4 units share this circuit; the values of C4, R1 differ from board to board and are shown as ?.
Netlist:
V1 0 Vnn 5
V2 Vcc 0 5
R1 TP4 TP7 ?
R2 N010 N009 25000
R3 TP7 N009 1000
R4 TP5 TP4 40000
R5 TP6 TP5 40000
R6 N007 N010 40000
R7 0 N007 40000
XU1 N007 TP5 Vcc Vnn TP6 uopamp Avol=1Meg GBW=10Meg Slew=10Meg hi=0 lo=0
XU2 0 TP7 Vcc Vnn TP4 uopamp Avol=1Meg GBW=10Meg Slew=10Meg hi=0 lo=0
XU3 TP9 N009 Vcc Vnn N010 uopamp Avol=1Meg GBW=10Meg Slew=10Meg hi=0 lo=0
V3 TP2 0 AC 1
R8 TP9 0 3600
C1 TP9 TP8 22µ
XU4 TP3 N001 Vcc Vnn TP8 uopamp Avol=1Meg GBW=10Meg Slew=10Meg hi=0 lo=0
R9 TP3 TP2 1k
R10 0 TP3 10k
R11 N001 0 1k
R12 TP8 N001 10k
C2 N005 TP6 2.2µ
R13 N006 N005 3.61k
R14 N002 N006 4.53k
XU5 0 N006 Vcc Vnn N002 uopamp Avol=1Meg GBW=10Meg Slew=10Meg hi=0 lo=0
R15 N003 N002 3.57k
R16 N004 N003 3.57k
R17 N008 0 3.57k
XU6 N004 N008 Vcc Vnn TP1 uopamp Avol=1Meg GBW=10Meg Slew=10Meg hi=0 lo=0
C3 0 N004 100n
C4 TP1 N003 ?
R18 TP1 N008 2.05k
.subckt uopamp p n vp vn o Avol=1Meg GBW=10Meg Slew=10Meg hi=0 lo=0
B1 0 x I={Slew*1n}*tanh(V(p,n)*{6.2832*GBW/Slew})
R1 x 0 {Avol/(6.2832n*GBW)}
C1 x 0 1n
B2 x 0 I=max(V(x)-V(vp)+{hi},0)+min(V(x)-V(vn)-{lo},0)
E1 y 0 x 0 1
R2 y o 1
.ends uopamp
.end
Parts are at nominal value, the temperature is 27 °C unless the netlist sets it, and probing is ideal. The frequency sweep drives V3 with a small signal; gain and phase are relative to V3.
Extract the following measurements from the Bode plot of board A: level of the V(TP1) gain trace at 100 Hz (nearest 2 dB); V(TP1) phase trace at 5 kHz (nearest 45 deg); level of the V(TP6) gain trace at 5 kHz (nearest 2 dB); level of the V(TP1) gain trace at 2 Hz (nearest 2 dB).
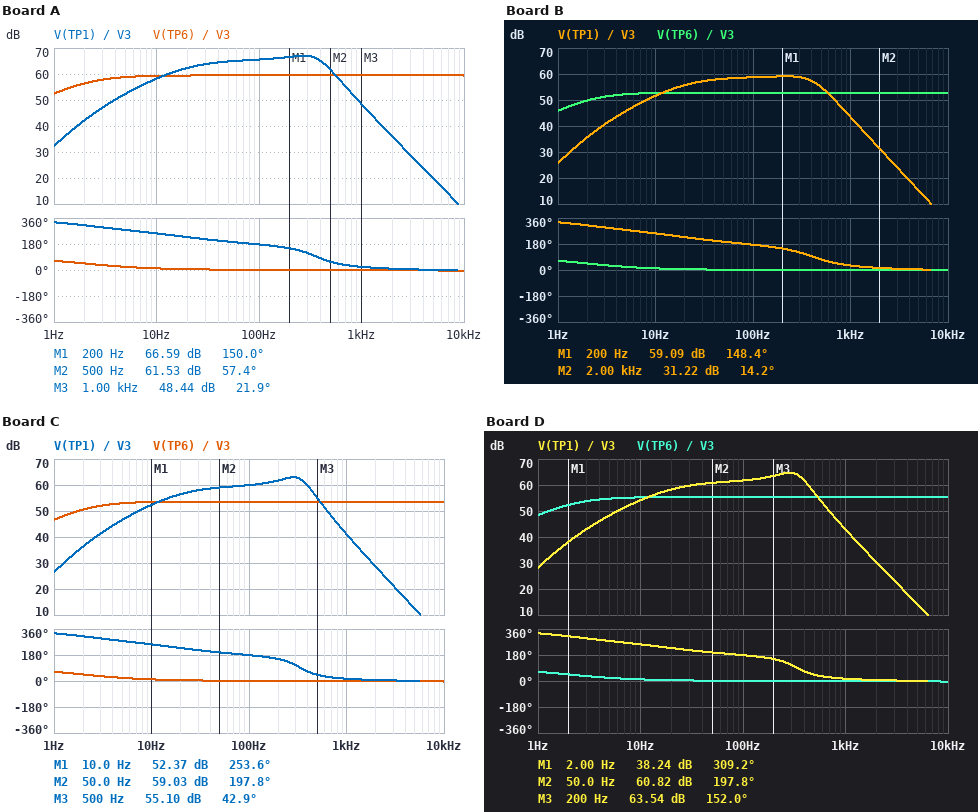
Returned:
66 dB
0 deg
60 dB
42 dB
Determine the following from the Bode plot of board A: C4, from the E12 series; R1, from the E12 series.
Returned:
150 nF
68 kΩ
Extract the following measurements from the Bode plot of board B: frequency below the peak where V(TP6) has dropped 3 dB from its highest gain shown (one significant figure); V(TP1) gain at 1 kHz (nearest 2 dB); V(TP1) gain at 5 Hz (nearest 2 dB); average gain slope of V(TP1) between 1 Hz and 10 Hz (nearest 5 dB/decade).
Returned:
2 Hz
44 dB
46 dB
25 dB/decade
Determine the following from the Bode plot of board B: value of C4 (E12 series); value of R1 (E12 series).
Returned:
120 nF
18 kΩ
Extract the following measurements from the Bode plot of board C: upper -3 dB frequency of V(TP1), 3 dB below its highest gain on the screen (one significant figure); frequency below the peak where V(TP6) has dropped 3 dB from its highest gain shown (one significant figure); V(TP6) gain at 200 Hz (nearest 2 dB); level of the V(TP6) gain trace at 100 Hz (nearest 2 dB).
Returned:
400 Hz
2 Hz
54 dB
54 dB
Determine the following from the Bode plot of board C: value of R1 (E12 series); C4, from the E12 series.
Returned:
22 kΩ
180 nF
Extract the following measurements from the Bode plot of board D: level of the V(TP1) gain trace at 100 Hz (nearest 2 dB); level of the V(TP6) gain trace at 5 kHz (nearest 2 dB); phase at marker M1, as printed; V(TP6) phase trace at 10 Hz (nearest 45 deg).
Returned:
62 dB
56 dB
309.2 deg
0 deg
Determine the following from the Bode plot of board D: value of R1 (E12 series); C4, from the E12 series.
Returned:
33 kΩ
180 nF
